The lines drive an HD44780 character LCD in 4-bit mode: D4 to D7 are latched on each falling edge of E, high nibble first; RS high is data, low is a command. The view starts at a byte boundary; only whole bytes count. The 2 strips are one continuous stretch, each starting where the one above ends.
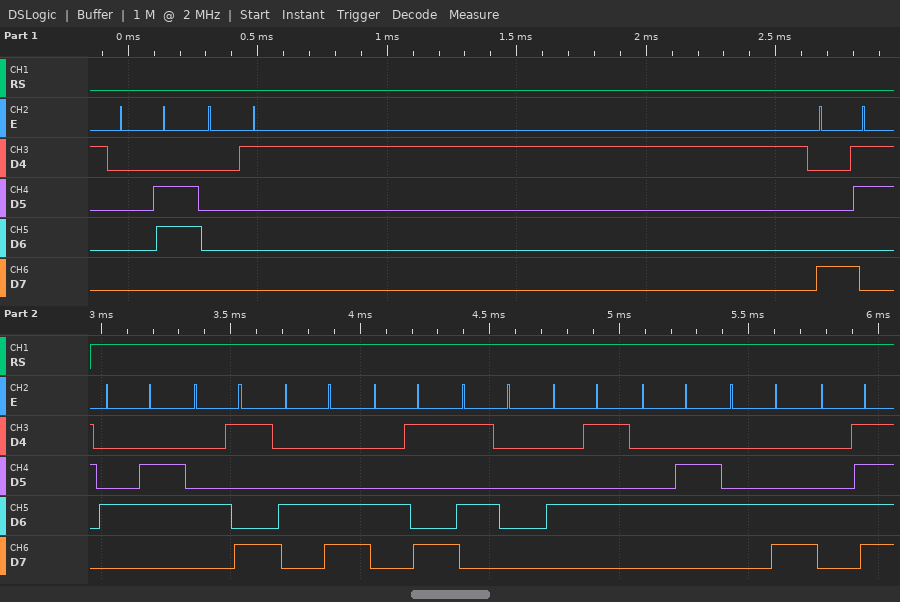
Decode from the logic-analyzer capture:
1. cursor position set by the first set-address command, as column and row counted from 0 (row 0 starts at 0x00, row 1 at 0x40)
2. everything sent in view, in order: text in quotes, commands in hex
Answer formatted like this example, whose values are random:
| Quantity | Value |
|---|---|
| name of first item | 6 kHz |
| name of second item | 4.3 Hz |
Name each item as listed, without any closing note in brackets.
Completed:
| Quantity | Value |
|---|---|
| cursor position set by the first set-address command, as column and row counted from 0 | column 3, row 0 |
| everything sent in view, in order: text in quotes, commands in hex | 0x06 0x01 0x83 "FILIPEFLO" |
